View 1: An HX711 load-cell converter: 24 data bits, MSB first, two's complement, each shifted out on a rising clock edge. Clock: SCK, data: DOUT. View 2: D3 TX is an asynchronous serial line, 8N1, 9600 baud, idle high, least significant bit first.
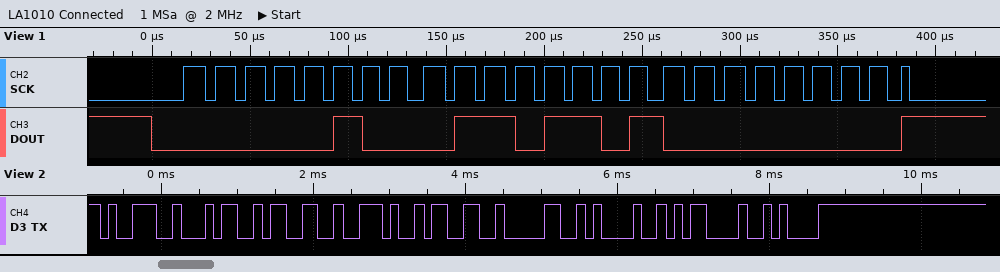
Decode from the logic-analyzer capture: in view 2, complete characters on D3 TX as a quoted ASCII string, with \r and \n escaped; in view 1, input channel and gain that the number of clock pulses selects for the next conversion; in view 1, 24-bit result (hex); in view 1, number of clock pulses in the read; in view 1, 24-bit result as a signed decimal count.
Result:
"943.30!\r\n"
channel A, gain 128
0x046D00
25
290048
